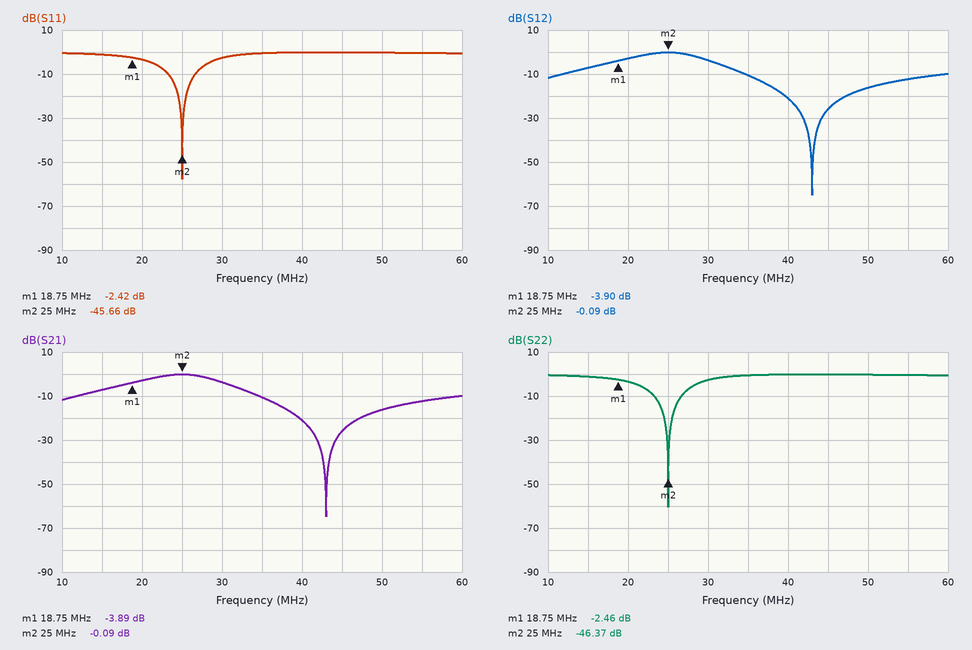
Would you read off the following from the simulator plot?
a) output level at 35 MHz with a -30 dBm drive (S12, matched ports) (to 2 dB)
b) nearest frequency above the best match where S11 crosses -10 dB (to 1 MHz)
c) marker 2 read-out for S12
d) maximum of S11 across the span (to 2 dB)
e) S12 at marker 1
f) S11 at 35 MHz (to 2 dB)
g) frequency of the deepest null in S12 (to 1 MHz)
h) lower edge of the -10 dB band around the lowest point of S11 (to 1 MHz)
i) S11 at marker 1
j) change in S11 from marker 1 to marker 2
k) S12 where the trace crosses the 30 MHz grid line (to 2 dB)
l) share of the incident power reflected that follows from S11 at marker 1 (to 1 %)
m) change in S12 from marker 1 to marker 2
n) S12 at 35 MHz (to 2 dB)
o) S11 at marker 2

-40 dBm
27 MHz
-0.09 dB
0 dB
-3.90 dB
0 dB
43 MHz
23 MHz
-2.42 dB
-43.24 dB
-4 dB
57 %
3.81 dB
-10 dB
-45.66 dB
